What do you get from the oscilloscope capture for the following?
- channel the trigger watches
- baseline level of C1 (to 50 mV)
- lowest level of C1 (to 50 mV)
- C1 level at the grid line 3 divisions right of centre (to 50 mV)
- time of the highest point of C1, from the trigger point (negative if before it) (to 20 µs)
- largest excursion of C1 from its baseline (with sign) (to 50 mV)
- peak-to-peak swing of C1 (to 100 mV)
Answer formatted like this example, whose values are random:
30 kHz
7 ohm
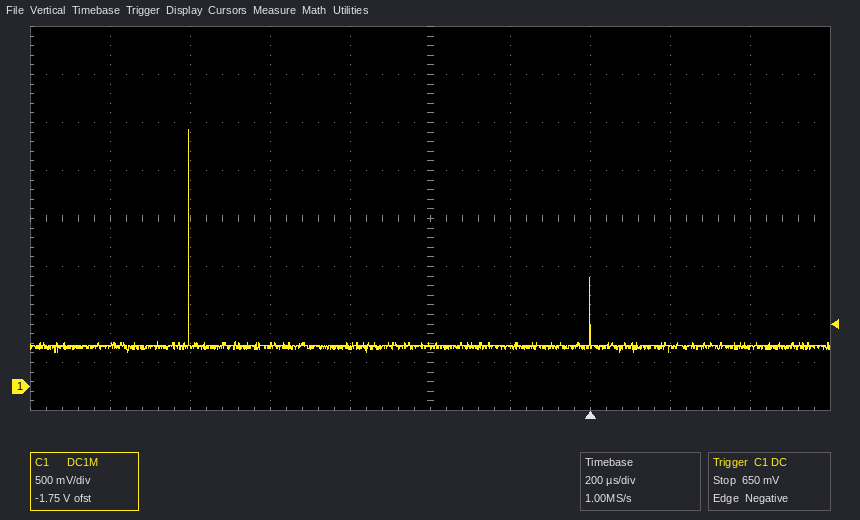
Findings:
C1
400 mV
350 mV
400 mV
-1.00 ms
+2.25 V
2.30 V
